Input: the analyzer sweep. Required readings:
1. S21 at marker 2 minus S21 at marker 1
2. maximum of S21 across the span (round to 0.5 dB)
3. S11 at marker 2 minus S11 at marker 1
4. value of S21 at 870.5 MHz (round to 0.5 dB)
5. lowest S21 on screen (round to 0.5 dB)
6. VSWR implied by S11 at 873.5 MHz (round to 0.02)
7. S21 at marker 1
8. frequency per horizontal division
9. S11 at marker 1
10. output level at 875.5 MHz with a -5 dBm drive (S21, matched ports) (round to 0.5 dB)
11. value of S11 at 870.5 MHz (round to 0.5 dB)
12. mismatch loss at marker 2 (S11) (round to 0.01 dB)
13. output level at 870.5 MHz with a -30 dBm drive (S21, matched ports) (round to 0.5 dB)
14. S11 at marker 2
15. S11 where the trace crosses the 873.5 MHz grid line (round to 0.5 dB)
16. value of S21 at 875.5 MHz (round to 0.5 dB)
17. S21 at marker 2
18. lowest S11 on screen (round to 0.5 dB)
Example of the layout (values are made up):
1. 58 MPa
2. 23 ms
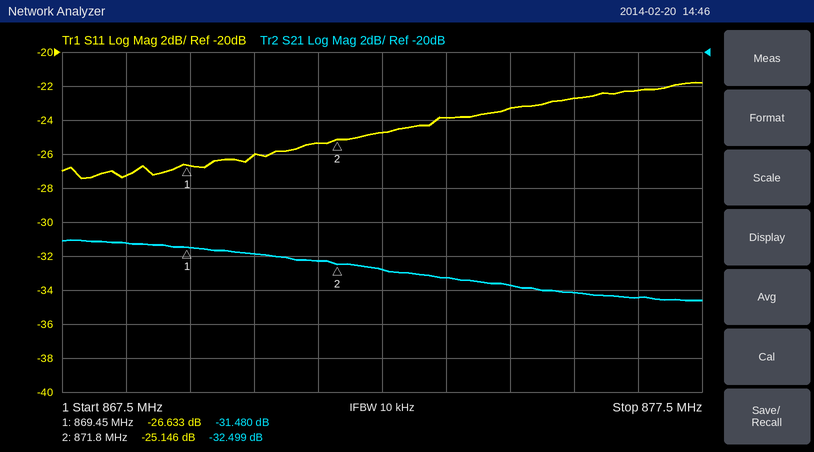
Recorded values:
1. -1.019 dB
2. -31.0 dB
3. 1.487 dB
4. -32.0 dB
5. -34.5 dB
6. 1.14
7. -31.480 dB
8. 1 MHz
9. -26.633 dB
10. -39.0 dBm
11. -26.0 dB
12. 0.01 dB
13. -62.0 dBm
14. -25.146 dB
15. -24.0 dB
16. -34.0 dB
17. -32.499 dB
18. -27.5 dB
